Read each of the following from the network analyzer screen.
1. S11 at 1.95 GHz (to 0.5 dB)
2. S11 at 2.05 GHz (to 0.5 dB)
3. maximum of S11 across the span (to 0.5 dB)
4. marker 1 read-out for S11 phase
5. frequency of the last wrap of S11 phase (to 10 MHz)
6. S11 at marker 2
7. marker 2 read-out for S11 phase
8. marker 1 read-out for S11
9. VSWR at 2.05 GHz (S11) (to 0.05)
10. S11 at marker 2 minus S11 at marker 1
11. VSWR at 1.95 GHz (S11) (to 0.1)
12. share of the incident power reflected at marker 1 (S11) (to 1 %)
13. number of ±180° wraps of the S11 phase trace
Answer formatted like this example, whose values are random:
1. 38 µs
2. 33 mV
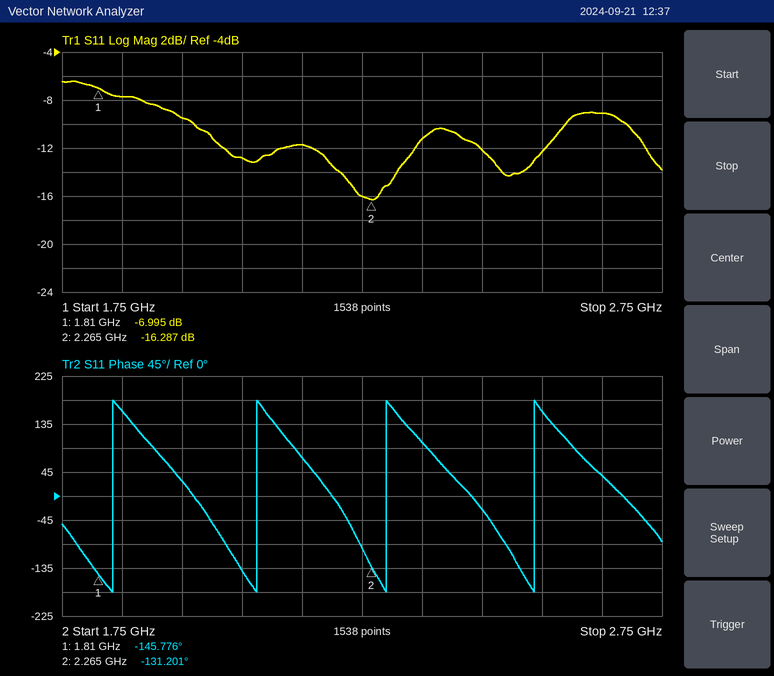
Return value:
1. -9.5 dB
2. -13.0 dB
3. -6.5 dB
4. -145.776°
5. 2.54 GHz
6. -16.287 dB
7. -131.201°
8. -6.995 dB
9. 1.60
10. -9.292 dB
11. 2.0
12. 20 %
13. 4
